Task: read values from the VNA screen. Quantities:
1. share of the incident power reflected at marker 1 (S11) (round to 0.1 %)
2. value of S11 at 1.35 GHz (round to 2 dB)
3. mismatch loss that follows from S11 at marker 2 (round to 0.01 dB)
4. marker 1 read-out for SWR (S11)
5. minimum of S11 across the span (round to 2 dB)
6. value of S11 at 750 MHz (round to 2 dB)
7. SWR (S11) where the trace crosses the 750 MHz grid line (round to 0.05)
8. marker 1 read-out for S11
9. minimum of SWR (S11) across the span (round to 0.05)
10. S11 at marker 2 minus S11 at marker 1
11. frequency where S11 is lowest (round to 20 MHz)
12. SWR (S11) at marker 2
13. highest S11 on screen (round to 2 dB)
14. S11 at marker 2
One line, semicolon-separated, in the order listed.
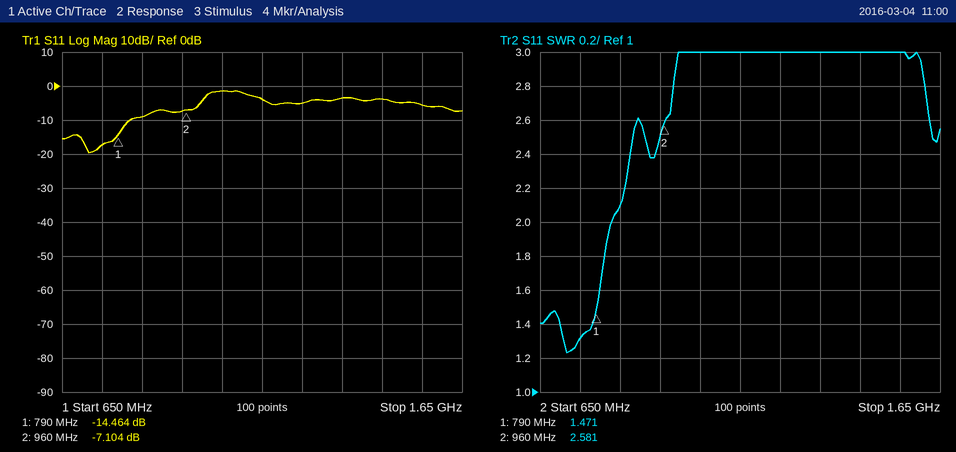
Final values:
3.6 %; -4 dB; 0.94 dB; 1.471; -20 dB; -18 dB; 1.30; -14.464 dB; 1.25; 7.360 dB; 720 MHz; 2.581; -2 dB; -7.104 dB
